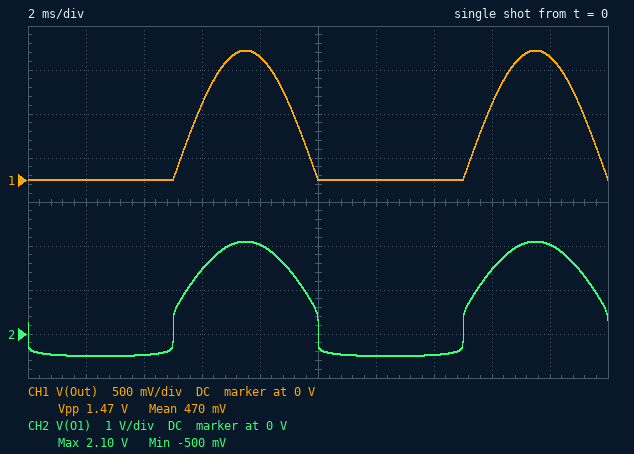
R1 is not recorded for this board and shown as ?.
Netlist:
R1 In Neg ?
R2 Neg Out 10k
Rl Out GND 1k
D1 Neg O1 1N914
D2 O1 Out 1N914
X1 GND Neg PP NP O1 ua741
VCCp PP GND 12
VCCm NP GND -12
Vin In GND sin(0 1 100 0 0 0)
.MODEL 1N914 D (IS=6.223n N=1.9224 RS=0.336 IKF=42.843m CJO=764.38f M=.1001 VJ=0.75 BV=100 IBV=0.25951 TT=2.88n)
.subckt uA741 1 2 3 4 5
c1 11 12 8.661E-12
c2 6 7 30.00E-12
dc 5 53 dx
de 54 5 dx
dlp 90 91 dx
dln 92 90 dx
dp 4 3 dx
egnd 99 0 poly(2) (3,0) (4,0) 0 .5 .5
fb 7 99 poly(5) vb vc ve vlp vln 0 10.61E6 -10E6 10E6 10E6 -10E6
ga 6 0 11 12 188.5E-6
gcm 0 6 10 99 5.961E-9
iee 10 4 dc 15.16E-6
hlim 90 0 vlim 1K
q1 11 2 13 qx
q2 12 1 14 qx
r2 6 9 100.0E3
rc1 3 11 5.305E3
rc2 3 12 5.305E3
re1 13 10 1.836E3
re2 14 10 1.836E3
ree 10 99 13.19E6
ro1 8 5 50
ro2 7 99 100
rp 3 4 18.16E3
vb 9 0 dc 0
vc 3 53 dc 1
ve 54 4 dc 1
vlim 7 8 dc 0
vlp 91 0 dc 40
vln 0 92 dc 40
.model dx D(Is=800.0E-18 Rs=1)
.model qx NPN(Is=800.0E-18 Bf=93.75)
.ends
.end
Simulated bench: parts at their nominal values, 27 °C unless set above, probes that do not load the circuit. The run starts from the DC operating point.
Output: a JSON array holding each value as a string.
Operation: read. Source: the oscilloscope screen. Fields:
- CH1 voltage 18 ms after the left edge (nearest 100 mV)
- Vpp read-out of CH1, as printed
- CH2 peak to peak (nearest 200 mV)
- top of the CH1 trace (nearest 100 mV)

["1.4 V", "1.47 V", "2.6 V", "1.5 V"]
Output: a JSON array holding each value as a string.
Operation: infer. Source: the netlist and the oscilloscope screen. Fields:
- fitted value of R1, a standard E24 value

["6.8 kΩ"]
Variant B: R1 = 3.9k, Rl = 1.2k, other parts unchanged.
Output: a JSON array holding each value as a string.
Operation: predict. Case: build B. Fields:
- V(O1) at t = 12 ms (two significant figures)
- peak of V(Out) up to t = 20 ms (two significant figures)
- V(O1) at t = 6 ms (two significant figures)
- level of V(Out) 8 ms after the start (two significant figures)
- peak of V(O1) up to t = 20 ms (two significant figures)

["-530 mV", "2.6 V", "2.1 V", "2.4 V", "3.2 V"]
